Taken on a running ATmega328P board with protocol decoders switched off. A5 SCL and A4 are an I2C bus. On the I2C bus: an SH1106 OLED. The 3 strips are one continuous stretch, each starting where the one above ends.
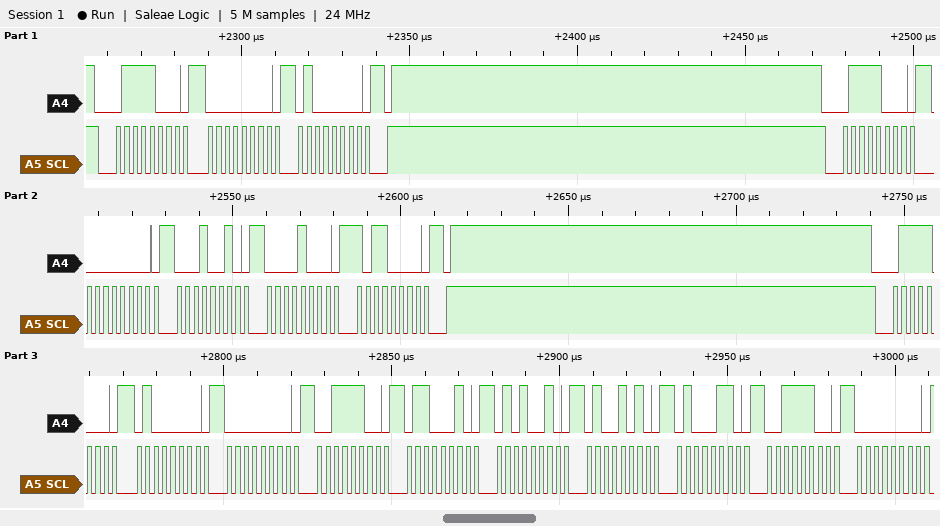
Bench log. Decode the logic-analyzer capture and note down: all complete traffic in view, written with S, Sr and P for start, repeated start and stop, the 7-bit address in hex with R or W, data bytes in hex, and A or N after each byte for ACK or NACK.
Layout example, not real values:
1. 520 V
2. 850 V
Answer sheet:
1. S 3CW A 00 A 40 A P S 3CW A 00 A 12 A 08 A B0 A P S 3CW A 40 A 00 A 3C A 62 A 52 A 4A A 46 A 3C A 00 A
